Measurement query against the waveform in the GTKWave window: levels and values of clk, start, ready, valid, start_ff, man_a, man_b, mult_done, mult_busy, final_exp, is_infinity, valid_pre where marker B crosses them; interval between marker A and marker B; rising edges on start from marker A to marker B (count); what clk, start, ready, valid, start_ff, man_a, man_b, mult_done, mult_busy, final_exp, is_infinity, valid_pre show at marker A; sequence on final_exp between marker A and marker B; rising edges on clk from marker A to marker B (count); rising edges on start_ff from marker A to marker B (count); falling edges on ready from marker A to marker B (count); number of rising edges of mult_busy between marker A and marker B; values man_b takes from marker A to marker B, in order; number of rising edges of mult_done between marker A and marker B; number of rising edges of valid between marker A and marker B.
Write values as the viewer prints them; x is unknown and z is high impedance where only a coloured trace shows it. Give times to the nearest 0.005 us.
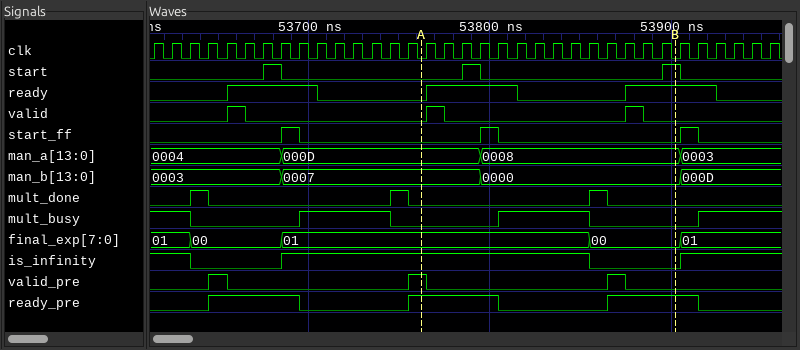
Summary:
clk=0, start=1, ready=1, valid=0, start_ff=0, man_a=0008, man_b=0000, mult_done=0, mult_busy=0, final_exp=00, is_infinity=0, valid_pre=0
0.14 us
2
clk=0, start=0, ready=0, valid=0, start_ff=0, man_a=000D, man_b=0007, mult_done=0, mult_busy=0, final_exp=01, is_infinity=1, valid_pre=1
01, 00
14
1
1
1
0007, 0000
1
2
